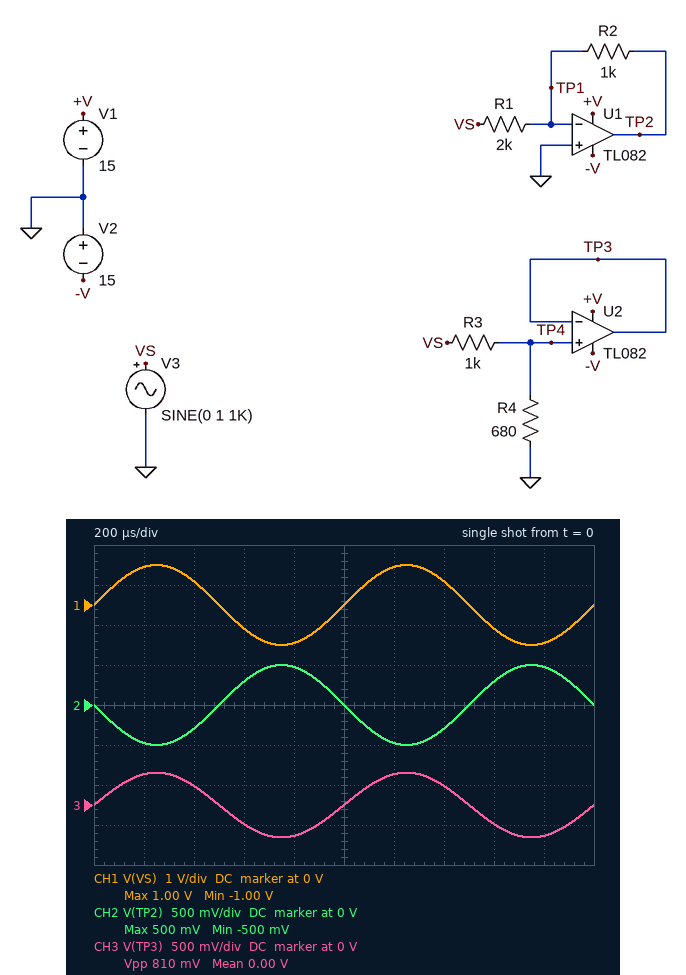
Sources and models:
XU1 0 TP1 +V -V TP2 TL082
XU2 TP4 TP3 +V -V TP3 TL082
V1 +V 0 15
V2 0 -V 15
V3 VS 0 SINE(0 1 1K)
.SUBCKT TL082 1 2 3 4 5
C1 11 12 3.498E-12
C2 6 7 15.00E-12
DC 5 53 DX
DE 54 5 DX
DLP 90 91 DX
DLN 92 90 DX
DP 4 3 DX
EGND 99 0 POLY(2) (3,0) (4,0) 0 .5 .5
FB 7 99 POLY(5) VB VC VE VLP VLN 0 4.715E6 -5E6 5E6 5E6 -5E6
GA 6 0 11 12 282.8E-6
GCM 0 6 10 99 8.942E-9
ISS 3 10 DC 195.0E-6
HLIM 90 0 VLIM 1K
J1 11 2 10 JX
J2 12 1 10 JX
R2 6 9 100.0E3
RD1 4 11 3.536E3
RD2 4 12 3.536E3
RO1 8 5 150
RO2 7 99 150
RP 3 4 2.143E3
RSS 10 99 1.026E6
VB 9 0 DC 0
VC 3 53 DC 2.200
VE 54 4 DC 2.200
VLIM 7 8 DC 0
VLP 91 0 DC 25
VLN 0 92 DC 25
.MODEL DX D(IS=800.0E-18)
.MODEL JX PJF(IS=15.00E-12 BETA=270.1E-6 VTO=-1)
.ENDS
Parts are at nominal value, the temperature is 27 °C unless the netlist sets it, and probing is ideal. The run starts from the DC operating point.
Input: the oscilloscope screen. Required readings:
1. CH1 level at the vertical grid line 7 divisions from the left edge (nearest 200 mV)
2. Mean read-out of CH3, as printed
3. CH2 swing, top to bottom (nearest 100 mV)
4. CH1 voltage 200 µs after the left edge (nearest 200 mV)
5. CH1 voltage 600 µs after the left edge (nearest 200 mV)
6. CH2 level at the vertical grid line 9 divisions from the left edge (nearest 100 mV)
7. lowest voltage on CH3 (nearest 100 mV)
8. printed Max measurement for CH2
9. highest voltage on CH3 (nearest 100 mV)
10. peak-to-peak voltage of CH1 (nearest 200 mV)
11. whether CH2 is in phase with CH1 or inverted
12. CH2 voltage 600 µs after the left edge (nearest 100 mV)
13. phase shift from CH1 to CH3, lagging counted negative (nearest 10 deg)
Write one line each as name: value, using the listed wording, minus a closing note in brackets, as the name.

CH1 level at the vertical grid line 7 divisions from the left edge: 600 mV
Mean read-out of CH3, as printed: 0.00 V
CH2 swing, top to bottom: 1.0 V
CH1 voltage 200 µs after the left edge: 1.0 V
CH1 voltage 600 µs after the left edge: -600 mV
CH2 level at the vertical grid line 9 divisions from the left edge: 500 mV
lowest voltage on CH3: -400 mV
printed Max measurement for CH2: 500 mV
highest voltage on CH3: 400 mV
peak-to-peak voltage of CH1: 2.0 V
whether CH2 is in phase with CH1 or inverted: inverted
CH2 voltage 600 µs after the left edge: 300 mV
phase shift from CH1 to CH3, lagging counted negative: 0 deg
